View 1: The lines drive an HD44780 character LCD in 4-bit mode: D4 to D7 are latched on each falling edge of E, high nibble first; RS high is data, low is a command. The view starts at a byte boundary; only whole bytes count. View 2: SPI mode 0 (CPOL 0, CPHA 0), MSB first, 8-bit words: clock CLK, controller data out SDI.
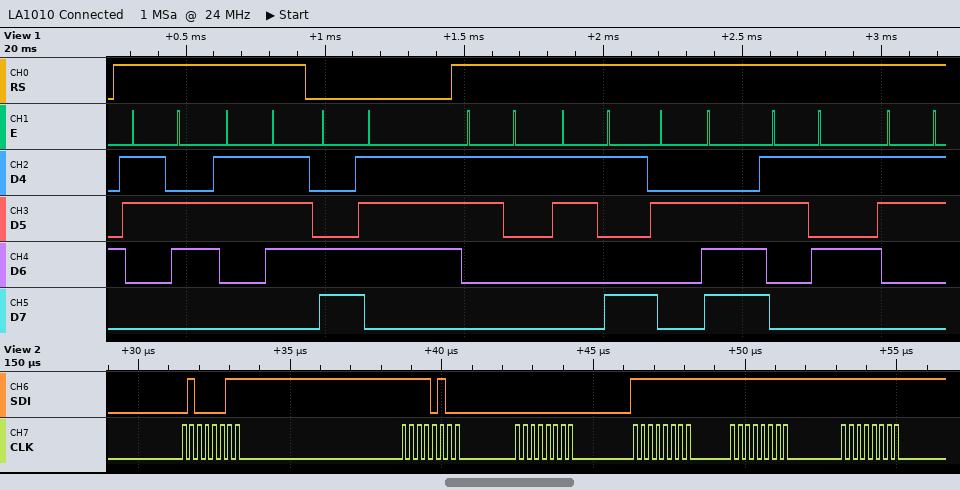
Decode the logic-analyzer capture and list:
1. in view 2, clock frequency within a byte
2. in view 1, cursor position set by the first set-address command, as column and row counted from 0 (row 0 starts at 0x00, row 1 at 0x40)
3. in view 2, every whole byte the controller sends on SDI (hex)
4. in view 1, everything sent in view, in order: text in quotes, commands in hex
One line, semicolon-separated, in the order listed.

4 MHz; column 7, row 1; 0x43 0xF4 0x00 0xFF 0xFF 0xFF; "67" 0xC7 "19.53"
